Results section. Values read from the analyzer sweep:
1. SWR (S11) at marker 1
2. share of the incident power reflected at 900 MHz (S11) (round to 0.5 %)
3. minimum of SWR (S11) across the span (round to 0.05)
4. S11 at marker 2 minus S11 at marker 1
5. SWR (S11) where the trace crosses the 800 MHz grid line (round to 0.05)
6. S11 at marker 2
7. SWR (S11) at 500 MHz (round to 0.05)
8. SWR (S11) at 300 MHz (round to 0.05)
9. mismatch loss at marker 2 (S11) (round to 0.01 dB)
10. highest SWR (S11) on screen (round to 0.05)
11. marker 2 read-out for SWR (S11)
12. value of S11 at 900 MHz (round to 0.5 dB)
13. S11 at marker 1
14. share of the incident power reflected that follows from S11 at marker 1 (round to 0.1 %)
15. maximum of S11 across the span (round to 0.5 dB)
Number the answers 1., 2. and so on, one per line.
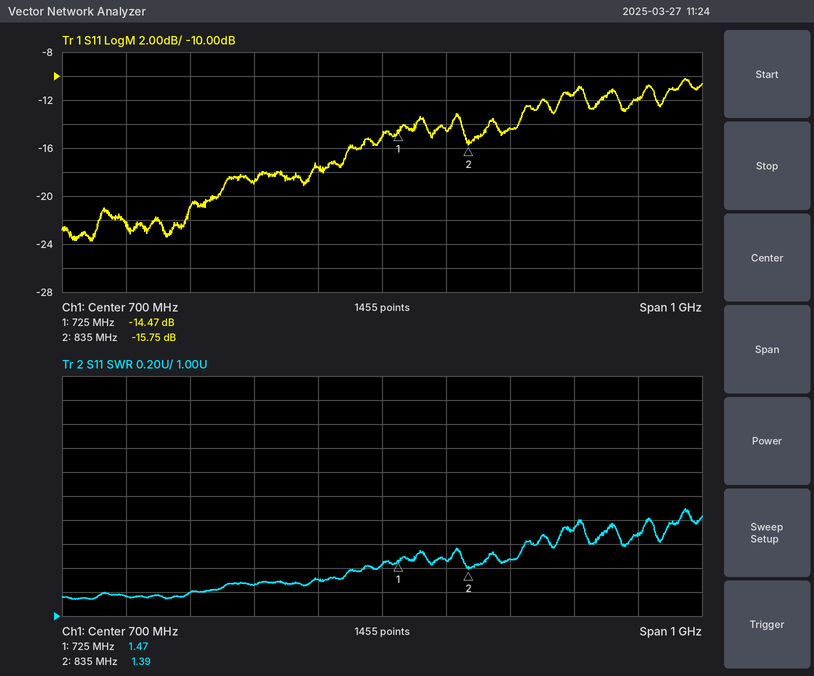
1. 1.47
2. 3.5 %
3. 1.15
4. -1.28 dB
5. 1.45
6. -15.75 dB
7. 1.25
8. 1.15
9. 0.12 dB
10. 1.90
11. 1.39
12. -14.5 dB
13. -14.47 dB
14. 3.6 %
15. -10.0 dB
